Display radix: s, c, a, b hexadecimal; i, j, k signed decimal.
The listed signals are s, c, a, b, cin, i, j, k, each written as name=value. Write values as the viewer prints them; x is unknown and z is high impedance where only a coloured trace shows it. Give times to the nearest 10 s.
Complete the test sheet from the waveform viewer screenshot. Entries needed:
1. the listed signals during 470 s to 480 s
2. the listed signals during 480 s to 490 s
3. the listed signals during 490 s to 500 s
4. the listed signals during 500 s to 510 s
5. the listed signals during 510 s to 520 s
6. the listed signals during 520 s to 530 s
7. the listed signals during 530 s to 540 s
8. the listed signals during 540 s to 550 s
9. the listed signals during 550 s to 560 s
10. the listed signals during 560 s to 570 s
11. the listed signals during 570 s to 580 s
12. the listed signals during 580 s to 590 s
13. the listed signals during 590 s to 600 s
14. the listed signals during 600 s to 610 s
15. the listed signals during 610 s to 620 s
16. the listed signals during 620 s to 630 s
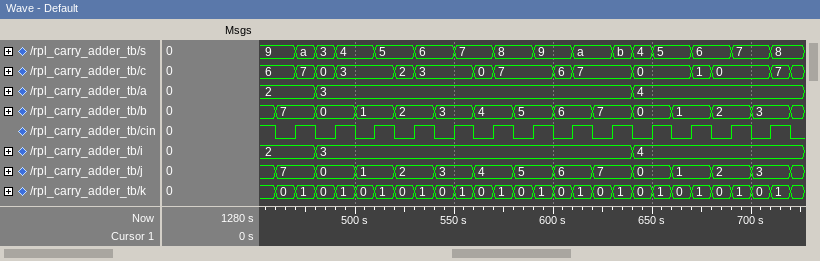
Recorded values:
s=a, c=7, a=2, b=7, cin=1, i=2, j=7, k=1
s=3, c=0, a=3, b=0, cin=0, i=3, j=0, k=0
s=4, c=3, a=3, b=0, cin=1, i=3, j=0, k=1
s=4, c=3, a=3, b=1, cin=0, i=3, j=1, k=0
s=5, c=3, a=3, b=1, cin=1, i=3, j=1, k=1
s=5, c=2, a=3, b=2, cin=0, i=3, j=2, k=0
s=6, c=3, a=3, b=2, cin=1, i=3, j=2, k=1
s=6, c=3, a=3, b=3, cin=0, i=3, j=3, k=0
s=7, c=3, a=3, b=3, cin=1, i=3, j=3, k=1
s=7, c=0, a=3, b=4, cin=0, i=3, j=4, k=0
s=8, c=7, a=3, b=4, cin=1, i=3, j=4, k=1
s=8, c=7, a=3, b=5, cin=0, i=3, j=5, k=0
s=9, c=7, a=3, b=5, cin=1, i=3, j=5, k=1
s=9, c=6, a=3, b=6, cin=0, i=3, j=6, k=0
s=a, c=7, a=3, b=6, cin=1, i=3, j=6, k=1
s=a, c=7, a=3, b=7, cin=0, i=3, j=7, k=0
